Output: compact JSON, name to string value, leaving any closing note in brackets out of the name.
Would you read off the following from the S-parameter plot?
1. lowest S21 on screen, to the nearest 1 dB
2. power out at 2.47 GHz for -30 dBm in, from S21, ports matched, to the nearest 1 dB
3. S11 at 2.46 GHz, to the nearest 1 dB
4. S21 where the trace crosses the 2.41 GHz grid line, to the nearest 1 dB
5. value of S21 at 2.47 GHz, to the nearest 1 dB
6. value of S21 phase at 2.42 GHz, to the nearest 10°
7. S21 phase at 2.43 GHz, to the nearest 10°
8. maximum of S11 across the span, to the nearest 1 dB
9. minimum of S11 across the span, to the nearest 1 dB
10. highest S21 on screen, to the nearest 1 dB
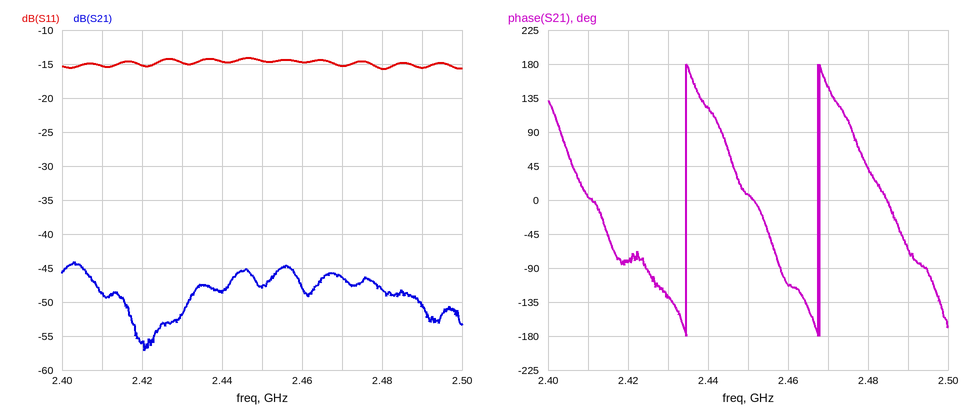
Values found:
{"lowest S21 on screen, to the nearest 1 dB": "-57 dB", "power out at 2.47 GHz for -30 dBm in, from S21, ports matched, to the nearest 1 dB": "-76 dBm", "S11 at 2.46 GHz, to the nearest 1 dB": "-15 dB", "S21 where the trace crosses the 2.41 GHz grid line, to the nearest 1 dB": "-49 dB", "value of S21 at 2.47 GHz, to the nearest 1 dB": "-46 dB", "value of S21 phase at 2.42 GHz, to the nearest 10°": "-80°", "S21 phase at 2.43 GHz, to the nearest 10°": "-130°", "maximum of S11 across the span, to the nearest 1 dB": "-14 dB", "minimum of S11 across the span, to the nearest 1 dB": "-16 dB", "highest S21 on screen, to the nearest 1 dB": "-44 dB"}
